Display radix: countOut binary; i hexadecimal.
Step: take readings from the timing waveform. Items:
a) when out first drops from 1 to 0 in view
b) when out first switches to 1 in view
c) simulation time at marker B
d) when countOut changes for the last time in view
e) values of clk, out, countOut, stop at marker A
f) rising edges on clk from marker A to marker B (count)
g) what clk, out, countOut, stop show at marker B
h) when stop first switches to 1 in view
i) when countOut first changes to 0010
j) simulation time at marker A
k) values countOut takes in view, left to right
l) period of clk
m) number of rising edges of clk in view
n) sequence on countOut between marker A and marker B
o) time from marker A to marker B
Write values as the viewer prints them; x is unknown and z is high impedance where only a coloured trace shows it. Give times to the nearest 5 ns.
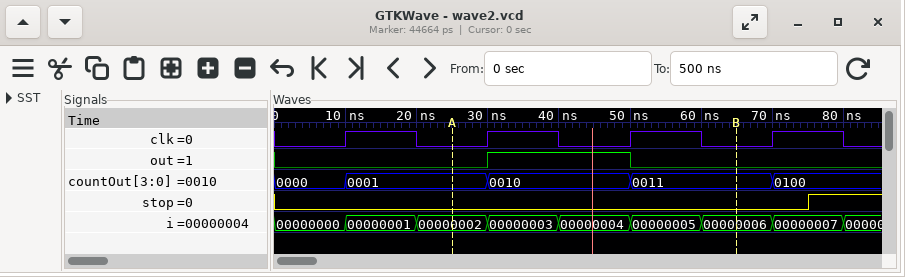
50 ns
30 ns
65 ns
70 ns
clk=0, out=0, countOut=0001, stop=0
2
clk=0, out=0, countOut=0011, stop=0
75 ns
30 ns
25 ns
0000, 0001, 0010, 0011, 0100
20 ns
4
0001, 0010, 0011
40 ns
